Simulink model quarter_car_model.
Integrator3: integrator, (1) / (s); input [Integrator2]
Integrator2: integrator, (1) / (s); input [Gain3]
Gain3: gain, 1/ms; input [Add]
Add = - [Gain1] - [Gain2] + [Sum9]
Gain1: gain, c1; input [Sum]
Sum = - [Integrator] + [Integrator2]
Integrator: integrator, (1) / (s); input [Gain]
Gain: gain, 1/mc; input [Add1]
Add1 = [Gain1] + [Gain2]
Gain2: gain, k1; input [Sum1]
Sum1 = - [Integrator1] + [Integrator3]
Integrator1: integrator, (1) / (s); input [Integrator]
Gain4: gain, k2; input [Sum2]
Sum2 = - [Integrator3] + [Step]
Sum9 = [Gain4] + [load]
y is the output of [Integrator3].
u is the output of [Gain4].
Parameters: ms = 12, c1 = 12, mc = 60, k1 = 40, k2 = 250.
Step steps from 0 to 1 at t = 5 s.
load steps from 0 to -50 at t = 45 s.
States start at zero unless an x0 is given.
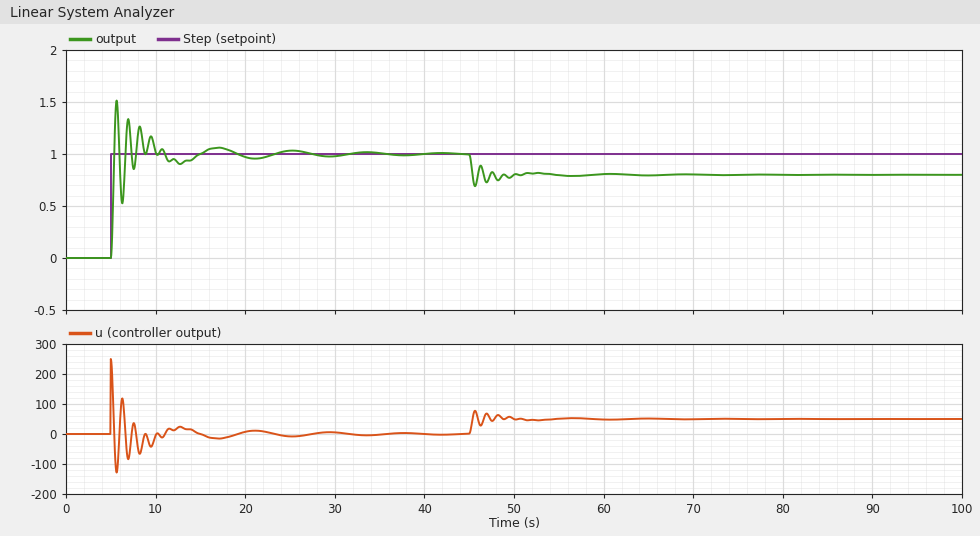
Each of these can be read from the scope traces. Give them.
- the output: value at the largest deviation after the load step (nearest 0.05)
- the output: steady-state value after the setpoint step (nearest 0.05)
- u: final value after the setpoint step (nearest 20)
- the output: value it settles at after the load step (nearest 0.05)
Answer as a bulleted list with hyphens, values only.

- 0.70
- 1.00
- 0
- 0.80
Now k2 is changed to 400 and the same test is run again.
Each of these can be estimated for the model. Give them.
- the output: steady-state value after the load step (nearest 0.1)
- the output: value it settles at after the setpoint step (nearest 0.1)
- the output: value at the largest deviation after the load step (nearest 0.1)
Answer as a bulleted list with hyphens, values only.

- 0.9
- 1.0
- 0.8
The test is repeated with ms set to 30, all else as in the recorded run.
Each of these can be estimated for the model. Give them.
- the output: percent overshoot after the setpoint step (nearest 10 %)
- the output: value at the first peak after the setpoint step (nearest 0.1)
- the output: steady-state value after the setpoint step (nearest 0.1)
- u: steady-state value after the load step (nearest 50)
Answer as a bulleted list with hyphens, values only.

- 60 %
- 1.6
- 1.0
- 50
